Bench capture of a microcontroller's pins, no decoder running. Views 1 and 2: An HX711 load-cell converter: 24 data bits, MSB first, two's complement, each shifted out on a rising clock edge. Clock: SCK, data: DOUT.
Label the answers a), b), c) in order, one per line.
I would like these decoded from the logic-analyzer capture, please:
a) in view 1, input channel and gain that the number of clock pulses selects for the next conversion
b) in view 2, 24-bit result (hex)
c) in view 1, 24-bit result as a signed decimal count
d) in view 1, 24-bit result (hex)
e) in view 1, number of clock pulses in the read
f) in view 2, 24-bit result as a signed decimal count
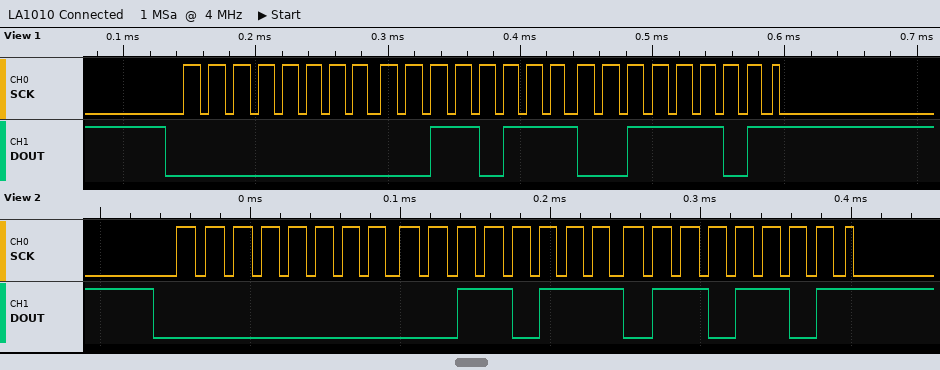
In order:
a) channel A, gain 128
b) 0x00376D
c) 14141
d) 0x00373D
e) 25
f) 14189
